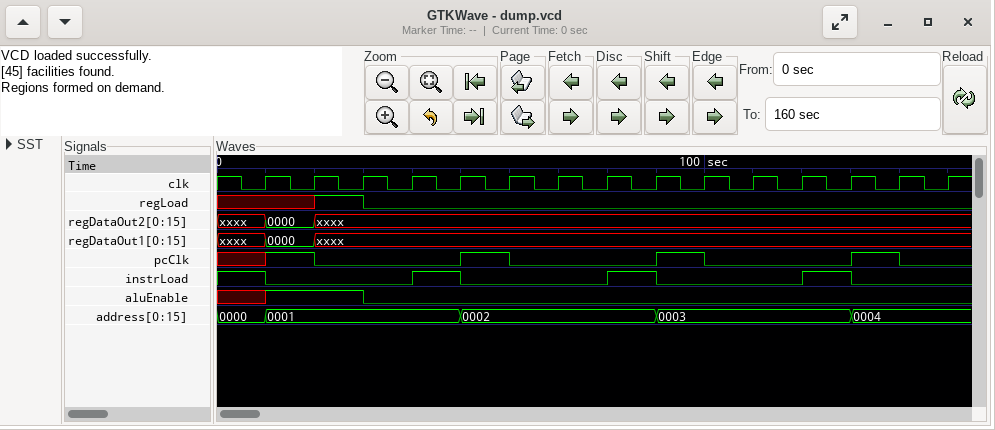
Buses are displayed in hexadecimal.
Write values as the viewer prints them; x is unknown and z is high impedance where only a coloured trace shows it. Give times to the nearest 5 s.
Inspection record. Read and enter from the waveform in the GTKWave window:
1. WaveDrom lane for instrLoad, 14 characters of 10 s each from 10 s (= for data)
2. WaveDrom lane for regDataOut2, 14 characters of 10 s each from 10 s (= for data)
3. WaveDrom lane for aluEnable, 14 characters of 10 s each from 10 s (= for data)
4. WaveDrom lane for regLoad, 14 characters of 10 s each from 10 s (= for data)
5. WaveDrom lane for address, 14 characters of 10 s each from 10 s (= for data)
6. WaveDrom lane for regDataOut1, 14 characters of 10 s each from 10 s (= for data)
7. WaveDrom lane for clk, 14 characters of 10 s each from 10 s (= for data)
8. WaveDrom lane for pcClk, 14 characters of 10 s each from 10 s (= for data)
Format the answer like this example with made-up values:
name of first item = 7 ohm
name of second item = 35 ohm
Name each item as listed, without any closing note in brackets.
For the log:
WaveDrom lane for instrLoad, 14 characters of 10 s each from 10 s = {name: 'instrLoad', wave: '0..10..10..10.'}
WaveDrom lane for regDataOut2, 14 characters of 10 s each from 10 s = {name: 'regDataOut2', wave: '=x............', data: '0000'}
WaveDrom lane for aluEnable, 14 characters of 10 s each from 10 s = {name: 'aluEnable', wave: '1.0...........'}
WaveDrom lane for regLoad, 14 characters of 10 s each from 10 s = {name: 'regLoad', wave: 'x10...........'}
WaveDrom lane for address, 14 characters of 10 s each from 10 s = {name: 'address', wave: '=...=...=...=.', data: '0001 0002 0003 0004'}
WaveDrom lane for regDataOut1, 14 characters of 10 s each from 10 s = {name: 'regDataOut1', wave: '=x............', data: '0000'}
WaveDrom lane for clk, 14 characters of 10 s each from 10 s = {name: 'clk', wave: 'p.............'}
WaveDrom lane for pcClk, 14 characters of 10 s each from 10 s = {name: 'pcClk', wave: '10..10..10..10'}
